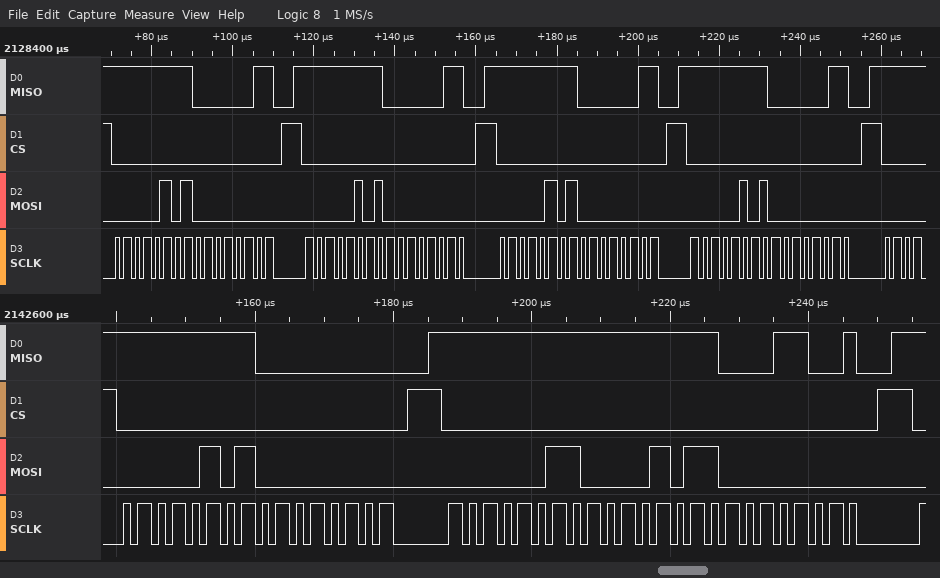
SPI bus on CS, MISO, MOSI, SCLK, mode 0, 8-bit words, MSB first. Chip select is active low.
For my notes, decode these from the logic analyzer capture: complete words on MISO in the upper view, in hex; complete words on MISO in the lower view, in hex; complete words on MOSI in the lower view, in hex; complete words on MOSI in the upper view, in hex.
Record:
FF, 03, FF, 03, FF, 03, FF, 03
FF, 00, FF, FF, 19
05, 00, 03, 0B, 00
05, 00, 05, 00, 05, 00, 05, 00
